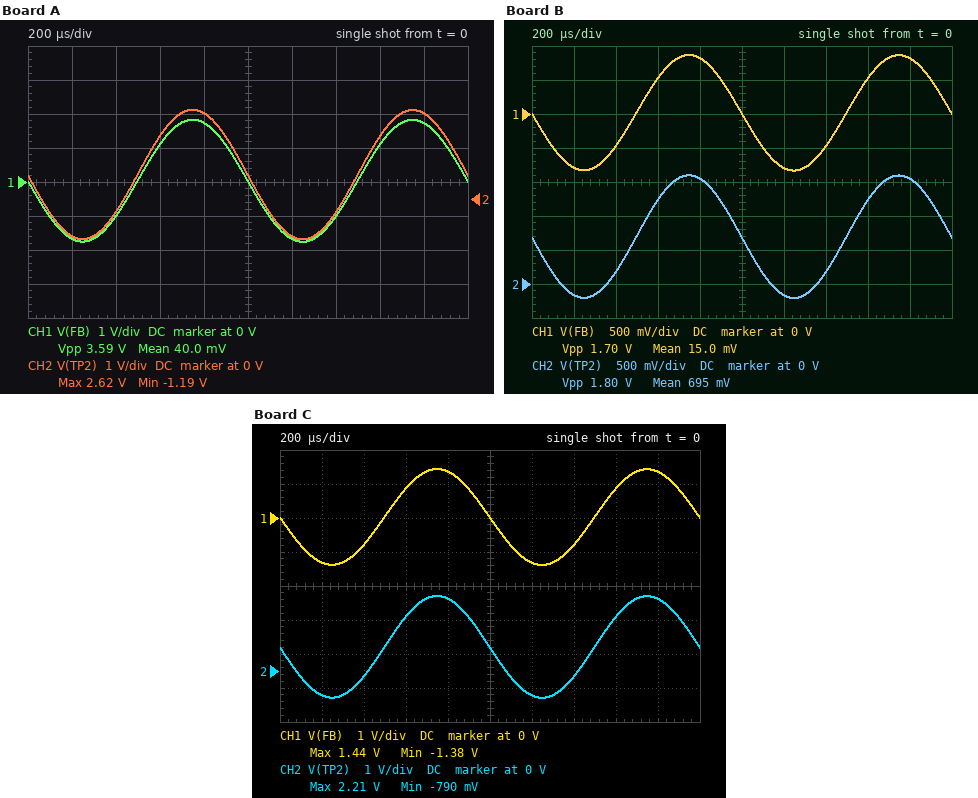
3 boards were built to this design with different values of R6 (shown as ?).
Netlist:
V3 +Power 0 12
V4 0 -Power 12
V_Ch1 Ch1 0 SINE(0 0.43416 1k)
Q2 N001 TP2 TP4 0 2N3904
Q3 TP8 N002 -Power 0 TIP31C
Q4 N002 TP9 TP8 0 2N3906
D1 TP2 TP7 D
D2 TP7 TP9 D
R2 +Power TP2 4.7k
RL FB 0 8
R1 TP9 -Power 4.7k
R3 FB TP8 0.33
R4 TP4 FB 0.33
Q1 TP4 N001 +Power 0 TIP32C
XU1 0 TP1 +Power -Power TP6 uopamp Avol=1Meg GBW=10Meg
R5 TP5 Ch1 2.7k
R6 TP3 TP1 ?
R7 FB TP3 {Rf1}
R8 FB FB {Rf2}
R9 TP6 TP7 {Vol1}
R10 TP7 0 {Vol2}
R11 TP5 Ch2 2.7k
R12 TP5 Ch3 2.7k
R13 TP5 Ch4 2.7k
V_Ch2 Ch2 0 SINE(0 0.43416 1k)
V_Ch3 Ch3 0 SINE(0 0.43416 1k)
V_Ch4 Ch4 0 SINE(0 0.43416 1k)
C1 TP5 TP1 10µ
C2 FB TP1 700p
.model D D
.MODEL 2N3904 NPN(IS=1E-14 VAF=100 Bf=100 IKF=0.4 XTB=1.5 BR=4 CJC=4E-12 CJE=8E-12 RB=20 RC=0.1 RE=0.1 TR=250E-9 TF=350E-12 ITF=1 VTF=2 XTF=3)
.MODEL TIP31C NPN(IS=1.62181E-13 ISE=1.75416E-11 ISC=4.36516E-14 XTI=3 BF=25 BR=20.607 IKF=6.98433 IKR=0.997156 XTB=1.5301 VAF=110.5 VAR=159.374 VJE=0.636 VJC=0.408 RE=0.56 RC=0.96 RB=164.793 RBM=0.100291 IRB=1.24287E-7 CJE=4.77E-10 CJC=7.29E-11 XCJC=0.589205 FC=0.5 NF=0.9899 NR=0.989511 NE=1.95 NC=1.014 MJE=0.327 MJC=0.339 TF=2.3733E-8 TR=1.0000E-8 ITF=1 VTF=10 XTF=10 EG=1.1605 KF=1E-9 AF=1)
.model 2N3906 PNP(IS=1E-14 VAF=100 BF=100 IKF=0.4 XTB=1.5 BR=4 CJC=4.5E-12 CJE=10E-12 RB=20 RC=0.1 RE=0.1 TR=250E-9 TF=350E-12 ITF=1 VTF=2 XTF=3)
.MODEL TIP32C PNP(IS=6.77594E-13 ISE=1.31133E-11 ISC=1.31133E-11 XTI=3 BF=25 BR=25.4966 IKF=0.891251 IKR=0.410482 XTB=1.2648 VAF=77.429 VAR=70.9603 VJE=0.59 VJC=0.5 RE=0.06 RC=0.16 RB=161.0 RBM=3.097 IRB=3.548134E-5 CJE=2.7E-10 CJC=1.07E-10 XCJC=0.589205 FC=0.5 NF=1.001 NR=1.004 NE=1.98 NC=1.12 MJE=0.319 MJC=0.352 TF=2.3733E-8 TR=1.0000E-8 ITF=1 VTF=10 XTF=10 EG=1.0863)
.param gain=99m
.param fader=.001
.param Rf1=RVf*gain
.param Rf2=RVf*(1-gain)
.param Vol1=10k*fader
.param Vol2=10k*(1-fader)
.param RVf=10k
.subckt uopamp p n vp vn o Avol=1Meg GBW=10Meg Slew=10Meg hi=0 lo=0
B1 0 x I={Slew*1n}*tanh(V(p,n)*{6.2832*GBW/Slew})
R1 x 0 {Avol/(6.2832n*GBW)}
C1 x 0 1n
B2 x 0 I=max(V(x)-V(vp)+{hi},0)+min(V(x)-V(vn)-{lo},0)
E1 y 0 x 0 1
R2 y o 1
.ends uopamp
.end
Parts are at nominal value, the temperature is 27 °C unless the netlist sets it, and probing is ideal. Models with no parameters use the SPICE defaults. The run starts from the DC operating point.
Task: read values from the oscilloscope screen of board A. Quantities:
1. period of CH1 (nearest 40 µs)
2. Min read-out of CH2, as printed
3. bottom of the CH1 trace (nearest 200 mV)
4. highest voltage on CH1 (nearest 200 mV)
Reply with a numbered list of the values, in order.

1. 1.00 ms
2. -1.19 V
3. -1.8 V
4. 1.8 V
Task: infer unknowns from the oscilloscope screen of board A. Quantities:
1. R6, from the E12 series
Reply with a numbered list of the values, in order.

1. 1.8 kΩ
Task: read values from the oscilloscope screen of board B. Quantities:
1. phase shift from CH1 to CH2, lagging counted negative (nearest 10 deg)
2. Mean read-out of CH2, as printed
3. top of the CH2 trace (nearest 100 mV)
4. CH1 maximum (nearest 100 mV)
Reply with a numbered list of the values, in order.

1. 0 deg
2. 695 mV
3. 1.6 V
4. 900 mV
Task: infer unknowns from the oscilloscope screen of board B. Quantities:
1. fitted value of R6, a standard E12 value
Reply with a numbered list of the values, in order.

1. 330 Ω
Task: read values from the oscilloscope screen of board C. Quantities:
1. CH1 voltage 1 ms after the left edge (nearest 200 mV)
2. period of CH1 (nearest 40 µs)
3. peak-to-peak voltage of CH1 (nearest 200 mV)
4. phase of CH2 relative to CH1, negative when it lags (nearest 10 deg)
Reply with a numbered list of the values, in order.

1. 0 V
2. 1.00 ms
3. 2.8 V
4. 0 deg
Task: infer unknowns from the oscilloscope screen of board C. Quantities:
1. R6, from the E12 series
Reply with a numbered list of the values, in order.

1. 1.2 kΩ
